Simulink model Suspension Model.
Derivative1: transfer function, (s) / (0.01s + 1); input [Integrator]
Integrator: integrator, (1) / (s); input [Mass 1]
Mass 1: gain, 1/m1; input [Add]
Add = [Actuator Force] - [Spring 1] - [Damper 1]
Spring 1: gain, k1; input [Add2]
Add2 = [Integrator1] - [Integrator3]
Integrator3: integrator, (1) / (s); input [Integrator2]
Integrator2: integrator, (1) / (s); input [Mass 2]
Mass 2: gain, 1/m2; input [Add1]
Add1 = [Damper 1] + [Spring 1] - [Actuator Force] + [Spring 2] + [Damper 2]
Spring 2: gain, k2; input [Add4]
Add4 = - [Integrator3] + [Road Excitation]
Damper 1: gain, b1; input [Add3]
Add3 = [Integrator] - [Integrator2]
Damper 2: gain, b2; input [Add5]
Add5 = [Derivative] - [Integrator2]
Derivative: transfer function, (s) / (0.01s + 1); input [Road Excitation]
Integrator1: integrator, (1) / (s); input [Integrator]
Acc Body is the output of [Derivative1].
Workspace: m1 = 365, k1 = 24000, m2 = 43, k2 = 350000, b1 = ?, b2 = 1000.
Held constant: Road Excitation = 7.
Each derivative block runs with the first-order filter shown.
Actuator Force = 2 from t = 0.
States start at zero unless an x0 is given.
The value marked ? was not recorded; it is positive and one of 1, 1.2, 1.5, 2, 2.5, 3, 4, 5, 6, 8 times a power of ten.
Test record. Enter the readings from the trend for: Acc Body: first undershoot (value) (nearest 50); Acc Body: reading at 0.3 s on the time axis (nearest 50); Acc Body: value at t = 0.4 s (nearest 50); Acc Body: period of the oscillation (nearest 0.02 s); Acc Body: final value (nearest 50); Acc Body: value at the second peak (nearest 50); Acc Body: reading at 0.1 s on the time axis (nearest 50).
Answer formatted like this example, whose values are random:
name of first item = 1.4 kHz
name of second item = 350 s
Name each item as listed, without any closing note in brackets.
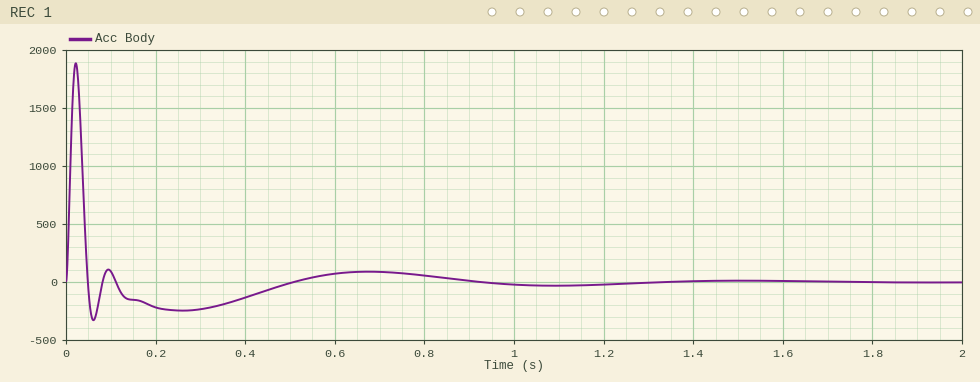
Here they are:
Acc Body: first undershoot (value) = -350
Acc Body: reading at 0.3 s on the time axis = -250
Acc Body: value at t = 0.4 s = -150
Acc Body: period of the oscillation = 0.08 s
Acc Body: final value = 0
Acc Body: value at the second peak = 100
Acc Body: reading at 0.1 s on the time axis = 100
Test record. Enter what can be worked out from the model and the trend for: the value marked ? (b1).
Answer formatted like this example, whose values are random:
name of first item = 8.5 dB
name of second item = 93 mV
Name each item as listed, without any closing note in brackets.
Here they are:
the value marked ? = 2000
